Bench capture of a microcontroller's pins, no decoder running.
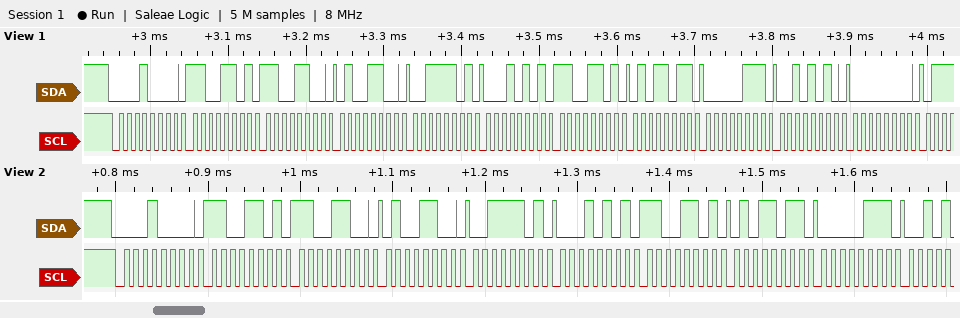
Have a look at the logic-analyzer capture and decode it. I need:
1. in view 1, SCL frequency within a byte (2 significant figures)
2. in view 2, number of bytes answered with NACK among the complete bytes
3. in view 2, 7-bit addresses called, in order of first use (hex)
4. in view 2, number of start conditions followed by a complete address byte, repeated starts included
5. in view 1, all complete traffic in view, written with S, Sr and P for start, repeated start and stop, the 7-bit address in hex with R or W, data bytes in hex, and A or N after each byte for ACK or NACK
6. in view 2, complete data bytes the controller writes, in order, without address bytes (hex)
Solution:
100 kHz
0
0x08
1
S 08W A CD A CC A 4C A 3D A 15 A CD A 5B A 07 A 2A A 00 A
CD CC 4C 3D 15 CD 5B 07
